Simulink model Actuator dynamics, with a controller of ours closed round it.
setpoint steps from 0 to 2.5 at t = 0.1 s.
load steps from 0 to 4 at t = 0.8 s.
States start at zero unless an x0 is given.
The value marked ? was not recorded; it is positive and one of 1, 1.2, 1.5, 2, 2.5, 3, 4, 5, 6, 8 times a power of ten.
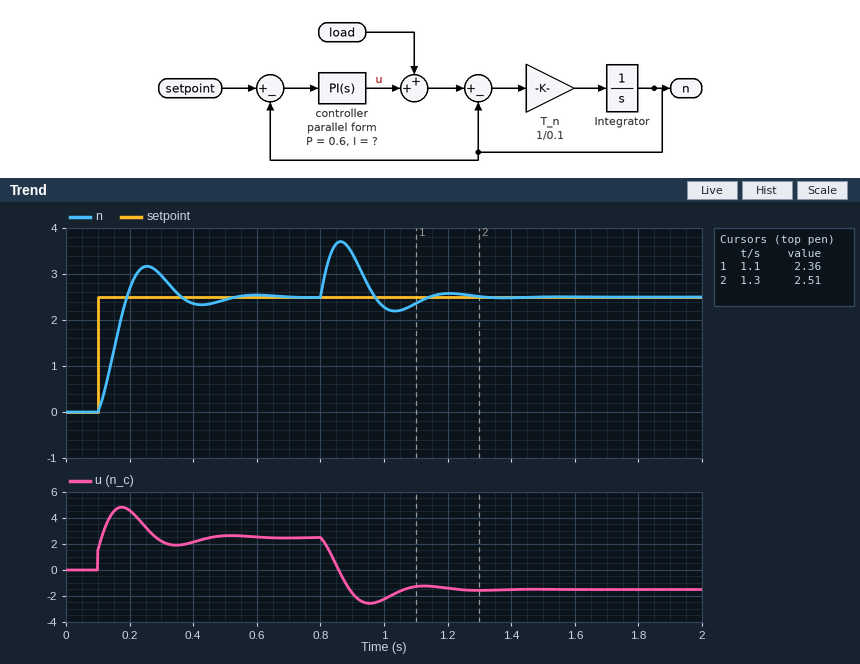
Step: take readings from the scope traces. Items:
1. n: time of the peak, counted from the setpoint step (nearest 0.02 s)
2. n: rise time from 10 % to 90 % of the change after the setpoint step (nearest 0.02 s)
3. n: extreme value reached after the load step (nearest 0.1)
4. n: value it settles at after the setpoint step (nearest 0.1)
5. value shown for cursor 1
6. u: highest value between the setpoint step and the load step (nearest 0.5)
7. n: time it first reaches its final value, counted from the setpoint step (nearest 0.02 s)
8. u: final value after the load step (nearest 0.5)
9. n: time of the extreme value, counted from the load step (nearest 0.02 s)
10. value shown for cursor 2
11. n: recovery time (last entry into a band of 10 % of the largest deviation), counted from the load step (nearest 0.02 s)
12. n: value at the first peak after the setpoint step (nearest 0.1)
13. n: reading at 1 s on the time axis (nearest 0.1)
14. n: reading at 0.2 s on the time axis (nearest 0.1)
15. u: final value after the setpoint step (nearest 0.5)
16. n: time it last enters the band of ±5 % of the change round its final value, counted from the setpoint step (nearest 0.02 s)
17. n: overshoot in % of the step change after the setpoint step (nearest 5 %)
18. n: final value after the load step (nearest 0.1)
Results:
0.16 s
0.06 s
3.7
2.5
2.36
5.0
0.10 s
-1.5
0.06 s
2.51
0.30 s
3.2
2.3
2.7
2.5
0.36 s
25 %
2.5
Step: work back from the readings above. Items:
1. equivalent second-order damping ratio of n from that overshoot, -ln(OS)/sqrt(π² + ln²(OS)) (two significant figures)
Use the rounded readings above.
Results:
0.40
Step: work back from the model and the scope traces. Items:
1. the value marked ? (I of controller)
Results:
40
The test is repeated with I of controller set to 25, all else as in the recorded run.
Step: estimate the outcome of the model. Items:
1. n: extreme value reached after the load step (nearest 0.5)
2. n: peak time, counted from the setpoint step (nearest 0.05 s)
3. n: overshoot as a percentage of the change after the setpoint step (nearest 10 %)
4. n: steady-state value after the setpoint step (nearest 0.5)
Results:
4.0
0.20 s
20 %
2.5
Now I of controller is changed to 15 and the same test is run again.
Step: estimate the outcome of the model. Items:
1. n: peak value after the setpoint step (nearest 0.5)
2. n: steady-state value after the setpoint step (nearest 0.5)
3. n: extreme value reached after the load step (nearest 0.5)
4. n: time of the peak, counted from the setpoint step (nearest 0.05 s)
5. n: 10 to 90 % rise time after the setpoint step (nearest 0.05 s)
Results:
2.5
2.5
4.0
0.30 s
0.15 s
